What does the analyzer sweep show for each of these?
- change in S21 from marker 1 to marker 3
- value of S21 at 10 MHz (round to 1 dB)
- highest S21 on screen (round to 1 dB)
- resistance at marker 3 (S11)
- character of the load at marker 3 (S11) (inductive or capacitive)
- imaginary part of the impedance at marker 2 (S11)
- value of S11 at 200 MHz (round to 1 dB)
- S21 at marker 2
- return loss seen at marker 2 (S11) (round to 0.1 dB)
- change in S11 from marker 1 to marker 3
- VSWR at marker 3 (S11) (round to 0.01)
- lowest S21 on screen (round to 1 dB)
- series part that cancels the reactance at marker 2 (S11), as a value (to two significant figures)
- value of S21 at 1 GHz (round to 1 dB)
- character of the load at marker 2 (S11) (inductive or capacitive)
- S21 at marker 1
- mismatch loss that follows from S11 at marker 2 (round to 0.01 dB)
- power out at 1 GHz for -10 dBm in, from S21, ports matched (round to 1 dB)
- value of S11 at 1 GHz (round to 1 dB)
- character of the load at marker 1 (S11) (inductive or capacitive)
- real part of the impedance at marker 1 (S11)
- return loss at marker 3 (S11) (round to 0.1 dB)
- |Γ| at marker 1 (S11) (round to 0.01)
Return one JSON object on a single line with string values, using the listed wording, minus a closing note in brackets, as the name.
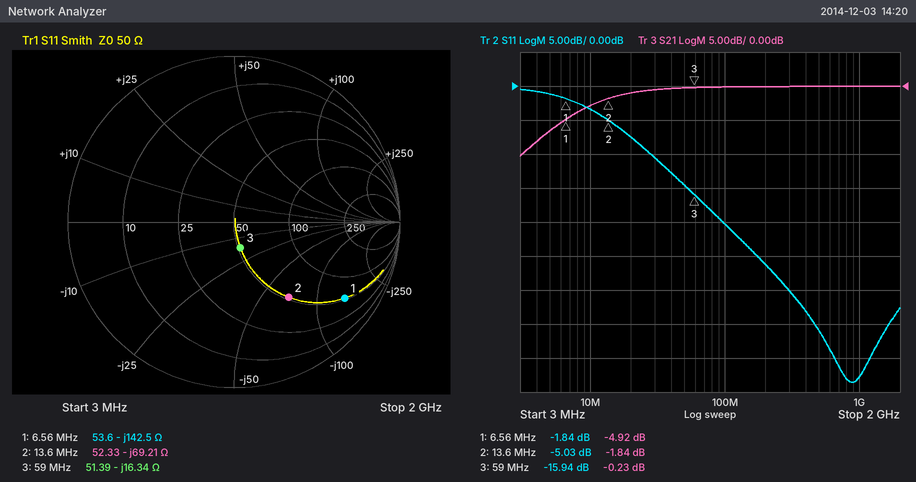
{"change in S21 from marker 1 to marker 3": "4.69 dB", "value of S21 at 10 MHz": "-3 dB", "highest S21 on screen": "0 dB", "resistance at marker 3": "51.39 Ω", "character of the load at marker 3 (S11)": "capacitive", "imaginary part of the impedance at marker 2": "-69.21 Ω", "value of S11 at 200 MHz": "-26 dB", "S21 at marker 2": "-1.84 dB", "return loss seen at marker 2 (S11)": "5.0 dB", "change in S11 from marker 1 to marker 3": "-14.10 dB", "VSWR at marker 3 (S11)": "1.38", "lowest S21 on screen": "-10 dB", "series part that cancels the reactance at marker 2 (S11), as a value": "810 nH", "value of S21 at 1 GHz": "0 dB", "character of the load at marker 2 (S11)": "capacitive", "S21 at marker 1": "-4.92 dB", "mismatch loss that follows from S11 at marker 2": "1.64 dB", "power out at 1 GHz for -10 dBm in, from S21, ports matched": "-10 dBm", "value of S11 at 1 GHz": "-43 dB", "character of the load at marker 1 (S11)": "capacitive", "real part of the impedance at marker 1": "53.6 Ω", "return loss at marker 3 (S11)": "15.9 dB", "|Γ| at marker 1 (S11)": "0.81"}
